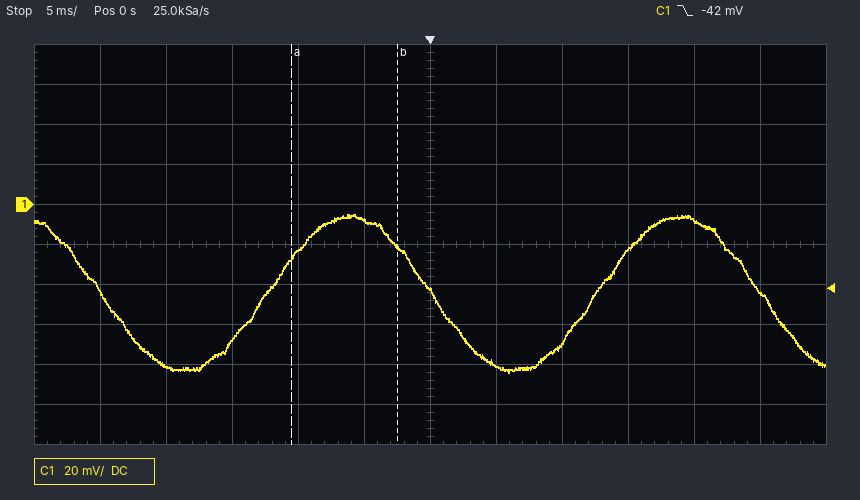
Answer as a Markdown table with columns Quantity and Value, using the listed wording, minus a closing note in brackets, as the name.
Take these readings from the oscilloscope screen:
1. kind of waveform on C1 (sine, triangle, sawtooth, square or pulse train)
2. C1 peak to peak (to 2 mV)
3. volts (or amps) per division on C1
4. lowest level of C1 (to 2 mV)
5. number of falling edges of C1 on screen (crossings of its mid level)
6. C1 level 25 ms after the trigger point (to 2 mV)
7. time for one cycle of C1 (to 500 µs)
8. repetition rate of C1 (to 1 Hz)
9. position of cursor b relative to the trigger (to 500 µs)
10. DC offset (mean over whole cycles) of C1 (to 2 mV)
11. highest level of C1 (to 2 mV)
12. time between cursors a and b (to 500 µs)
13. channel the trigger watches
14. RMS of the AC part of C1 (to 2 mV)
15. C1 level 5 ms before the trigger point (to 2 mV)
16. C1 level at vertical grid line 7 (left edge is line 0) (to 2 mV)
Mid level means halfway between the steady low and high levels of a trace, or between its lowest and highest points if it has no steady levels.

| Quantity | Value |
|---|---|
| kind of waveform on C1 | sine |
| C1 peak to peak | 80 mV |
| volts (or amps) per division on C1 | 20 mV |
| lowest level of C1 | -84 mV |
| number of falling edges of C1 on screen | 3 |
| C1 level 25 ms after the trigger point | -44 mV |
| time for one cycle of C1 | 25.0 ms |
| repetition rate of C1 | 40 Hz |
| position of cursor b relative to the trigger | -2.5 ms |
| DC offset (mean over whole cycles) of C1 | -44 mV |
| highest level of C1 | -4 mV |
| time between cursors a and b | 8.0 ms |
| channel the trigger watches | C1 |
| RMS of the AC part of C1 | 28 mV |
| C1 level 5 ms before the trigger point | -8 mV |
| C1 level at vertical grid line 7 (left edge is line 0) | -80 mV |
